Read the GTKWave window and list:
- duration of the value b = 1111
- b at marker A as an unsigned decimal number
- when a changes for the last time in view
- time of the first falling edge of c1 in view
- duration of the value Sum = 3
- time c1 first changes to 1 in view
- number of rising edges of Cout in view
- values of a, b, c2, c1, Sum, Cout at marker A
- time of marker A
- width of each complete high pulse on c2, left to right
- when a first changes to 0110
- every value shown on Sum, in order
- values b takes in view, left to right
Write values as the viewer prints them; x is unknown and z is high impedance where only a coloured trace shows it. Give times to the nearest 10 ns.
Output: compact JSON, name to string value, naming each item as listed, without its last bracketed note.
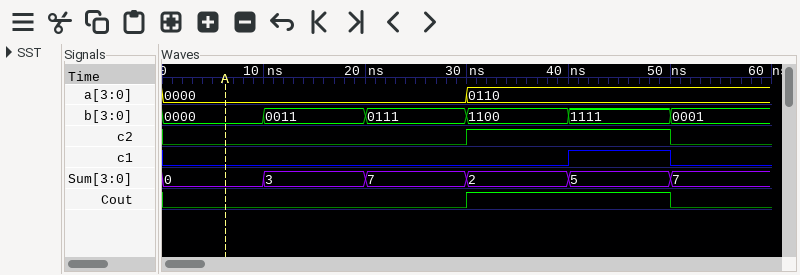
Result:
{"duration of the value b = 1111": "10 ns", "b at marker A as an unsigned decimal number": "0", "when a changes for the last time in view": "30 ns", "time of the first falling edge of c1 in view": "50 ns", "duration of the value Sum = 3": "10 ns", "time c1 first changes to 1 in view": "40 ns", "number of rising edges of Cout in view": "1", "values of a, b, c2, c1, Sum, Cout at marker A": "a=0000, b=0000, c2=0, c1=0, Sum=0, Cout=0", "time of marker A": "10 ns", "width of each complete high pulse on c2, left to right": "20 ns", "when a first changes to 0110": "30 ns", "every value shown on Sum, in order": "0, 3, 7, 2, 5, 7", "values b takes in view, left to right": "0000, 0011, 0111, 1100, 1111, 0001"}
